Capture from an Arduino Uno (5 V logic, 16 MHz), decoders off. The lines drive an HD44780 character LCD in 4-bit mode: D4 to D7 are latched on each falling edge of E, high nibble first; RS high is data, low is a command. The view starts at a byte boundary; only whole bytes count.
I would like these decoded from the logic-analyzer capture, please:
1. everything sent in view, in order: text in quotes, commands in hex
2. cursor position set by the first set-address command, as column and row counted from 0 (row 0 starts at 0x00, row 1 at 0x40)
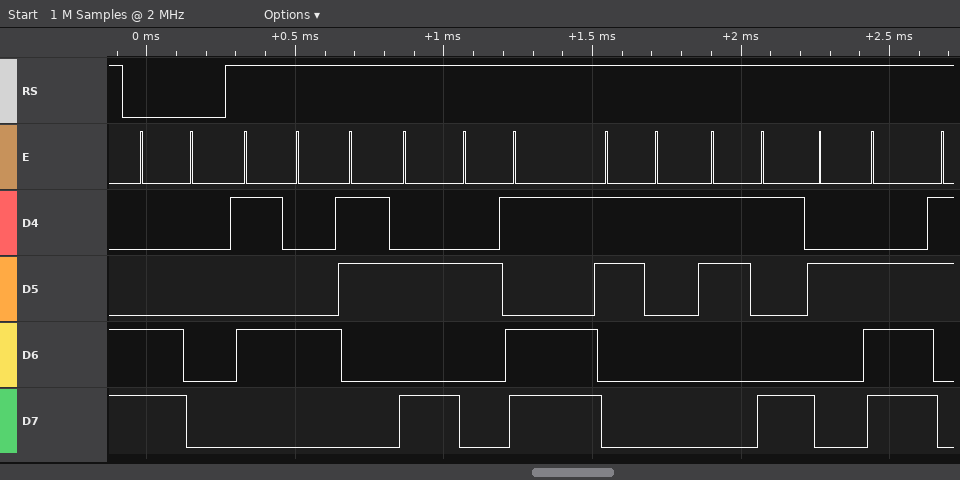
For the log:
0xC0 "T:-19."
column 0, row 1
